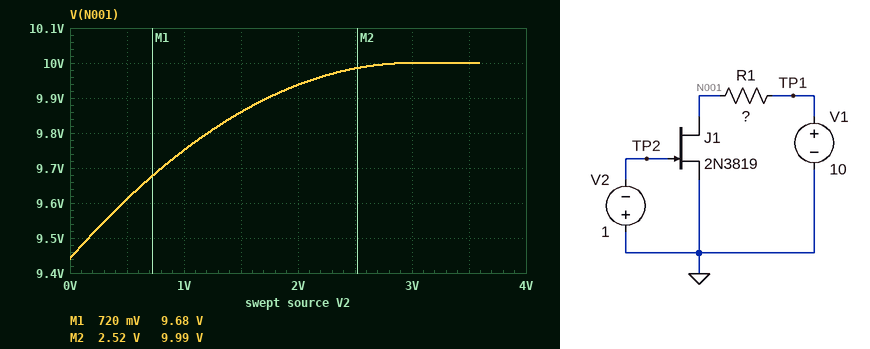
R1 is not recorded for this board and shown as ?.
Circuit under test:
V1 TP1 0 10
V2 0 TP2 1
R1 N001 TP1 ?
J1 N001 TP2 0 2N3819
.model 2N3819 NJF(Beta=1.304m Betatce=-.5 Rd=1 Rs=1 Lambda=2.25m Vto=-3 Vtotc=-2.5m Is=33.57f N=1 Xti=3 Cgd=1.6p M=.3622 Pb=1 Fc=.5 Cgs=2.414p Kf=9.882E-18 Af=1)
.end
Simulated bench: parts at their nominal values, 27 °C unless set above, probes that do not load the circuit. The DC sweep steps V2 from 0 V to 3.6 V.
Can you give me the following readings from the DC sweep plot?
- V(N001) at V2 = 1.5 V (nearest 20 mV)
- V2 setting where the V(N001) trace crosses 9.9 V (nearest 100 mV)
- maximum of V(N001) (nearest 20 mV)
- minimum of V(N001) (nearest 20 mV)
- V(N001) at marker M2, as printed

9.86 V
1.7 V
10.00 V
9.44 V
9.99 V
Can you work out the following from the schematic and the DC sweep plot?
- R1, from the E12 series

47 Ω
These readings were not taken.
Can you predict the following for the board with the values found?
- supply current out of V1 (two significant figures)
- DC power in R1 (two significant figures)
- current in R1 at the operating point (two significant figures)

5.3 mA
1.3 mW
5.3 mA
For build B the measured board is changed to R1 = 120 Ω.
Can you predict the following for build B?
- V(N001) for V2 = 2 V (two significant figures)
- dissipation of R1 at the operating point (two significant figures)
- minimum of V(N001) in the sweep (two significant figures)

9.8 V
3.4 mW
8.6 V
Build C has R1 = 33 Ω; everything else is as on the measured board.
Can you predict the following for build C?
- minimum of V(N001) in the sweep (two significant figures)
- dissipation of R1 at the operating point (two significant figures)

9.6 V
930 µW
